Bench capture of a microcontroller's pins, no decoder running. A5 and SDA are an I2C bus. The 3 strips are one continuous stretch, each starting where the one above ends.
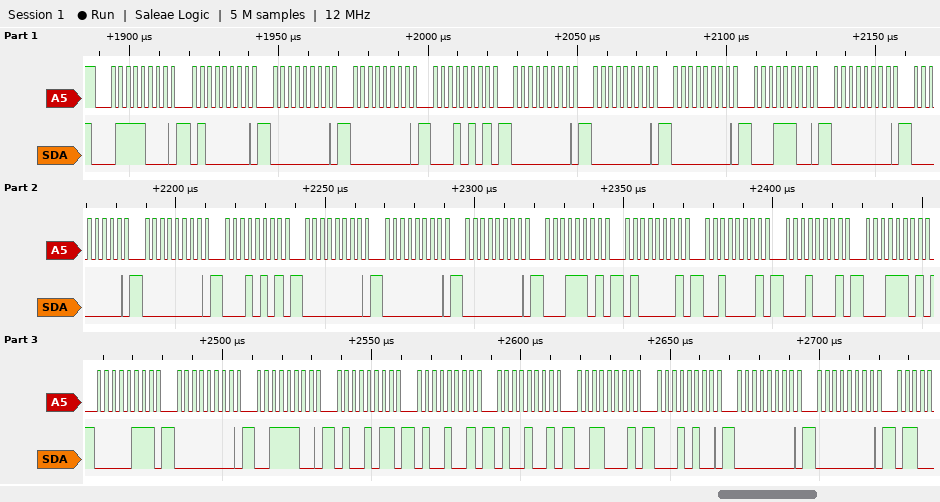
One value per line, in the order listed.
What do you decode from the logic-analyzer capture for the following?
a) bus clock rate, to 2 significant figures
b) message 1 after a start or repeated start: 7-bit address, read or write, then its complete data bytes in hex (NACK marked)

400 kHz
0x3C write: 40 00 00 15 00 00 00 1C 00 00 00 15 00 00 00 1D 41 21 11 1D 07 00 3C 4B 49 49 31 14 00 00
